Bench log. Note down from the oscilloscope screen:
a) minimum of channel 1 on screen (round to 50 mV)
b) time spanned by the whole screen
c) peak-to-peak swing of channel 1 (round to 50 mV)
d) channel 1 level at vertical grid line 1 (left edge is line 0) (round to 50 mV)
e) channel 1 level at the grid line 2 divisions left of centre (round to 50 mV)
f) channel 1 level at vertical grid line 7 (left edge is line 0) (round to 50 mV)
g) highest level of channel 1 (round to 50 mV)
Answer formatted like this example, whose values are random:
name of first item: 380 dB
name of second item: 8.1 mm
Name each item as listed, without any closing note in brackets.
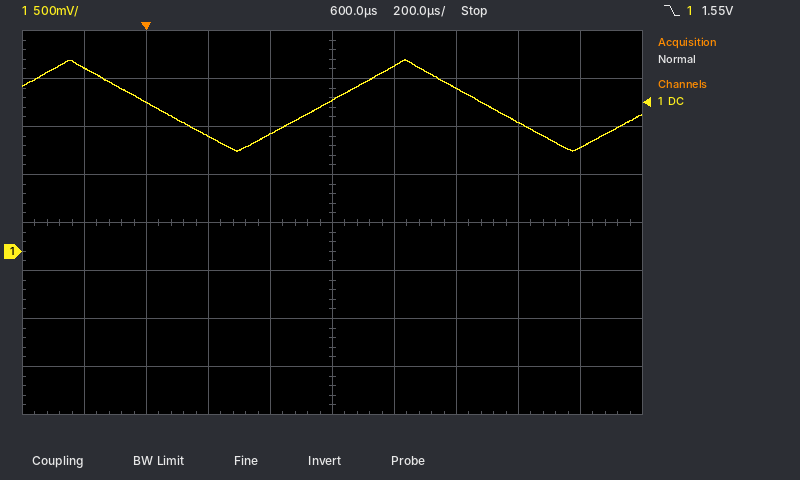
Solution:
minimum of channel 1 on screen: 1.05 V
time spanned by the whole screen: 2 ms
peak-to-peak swing of channel 1: 950 mV
channel 1 level at vertical grid line 1 (left edge is line 0): 1.90 V
channel 1 level at the grid line 2 divisions left of centre: 1.20 V
channel 1 level at vertical grid line 7 (left edge is line 0): 1.70 V
highest level of channel 1: 2.00 V
